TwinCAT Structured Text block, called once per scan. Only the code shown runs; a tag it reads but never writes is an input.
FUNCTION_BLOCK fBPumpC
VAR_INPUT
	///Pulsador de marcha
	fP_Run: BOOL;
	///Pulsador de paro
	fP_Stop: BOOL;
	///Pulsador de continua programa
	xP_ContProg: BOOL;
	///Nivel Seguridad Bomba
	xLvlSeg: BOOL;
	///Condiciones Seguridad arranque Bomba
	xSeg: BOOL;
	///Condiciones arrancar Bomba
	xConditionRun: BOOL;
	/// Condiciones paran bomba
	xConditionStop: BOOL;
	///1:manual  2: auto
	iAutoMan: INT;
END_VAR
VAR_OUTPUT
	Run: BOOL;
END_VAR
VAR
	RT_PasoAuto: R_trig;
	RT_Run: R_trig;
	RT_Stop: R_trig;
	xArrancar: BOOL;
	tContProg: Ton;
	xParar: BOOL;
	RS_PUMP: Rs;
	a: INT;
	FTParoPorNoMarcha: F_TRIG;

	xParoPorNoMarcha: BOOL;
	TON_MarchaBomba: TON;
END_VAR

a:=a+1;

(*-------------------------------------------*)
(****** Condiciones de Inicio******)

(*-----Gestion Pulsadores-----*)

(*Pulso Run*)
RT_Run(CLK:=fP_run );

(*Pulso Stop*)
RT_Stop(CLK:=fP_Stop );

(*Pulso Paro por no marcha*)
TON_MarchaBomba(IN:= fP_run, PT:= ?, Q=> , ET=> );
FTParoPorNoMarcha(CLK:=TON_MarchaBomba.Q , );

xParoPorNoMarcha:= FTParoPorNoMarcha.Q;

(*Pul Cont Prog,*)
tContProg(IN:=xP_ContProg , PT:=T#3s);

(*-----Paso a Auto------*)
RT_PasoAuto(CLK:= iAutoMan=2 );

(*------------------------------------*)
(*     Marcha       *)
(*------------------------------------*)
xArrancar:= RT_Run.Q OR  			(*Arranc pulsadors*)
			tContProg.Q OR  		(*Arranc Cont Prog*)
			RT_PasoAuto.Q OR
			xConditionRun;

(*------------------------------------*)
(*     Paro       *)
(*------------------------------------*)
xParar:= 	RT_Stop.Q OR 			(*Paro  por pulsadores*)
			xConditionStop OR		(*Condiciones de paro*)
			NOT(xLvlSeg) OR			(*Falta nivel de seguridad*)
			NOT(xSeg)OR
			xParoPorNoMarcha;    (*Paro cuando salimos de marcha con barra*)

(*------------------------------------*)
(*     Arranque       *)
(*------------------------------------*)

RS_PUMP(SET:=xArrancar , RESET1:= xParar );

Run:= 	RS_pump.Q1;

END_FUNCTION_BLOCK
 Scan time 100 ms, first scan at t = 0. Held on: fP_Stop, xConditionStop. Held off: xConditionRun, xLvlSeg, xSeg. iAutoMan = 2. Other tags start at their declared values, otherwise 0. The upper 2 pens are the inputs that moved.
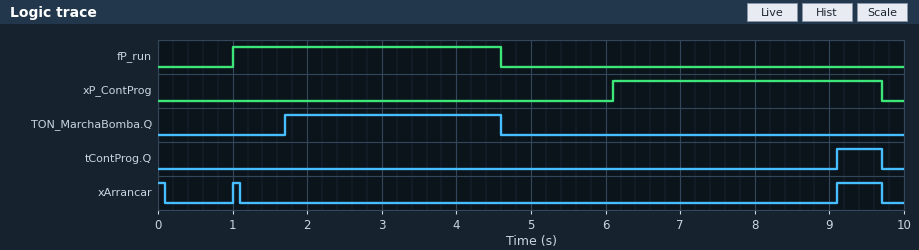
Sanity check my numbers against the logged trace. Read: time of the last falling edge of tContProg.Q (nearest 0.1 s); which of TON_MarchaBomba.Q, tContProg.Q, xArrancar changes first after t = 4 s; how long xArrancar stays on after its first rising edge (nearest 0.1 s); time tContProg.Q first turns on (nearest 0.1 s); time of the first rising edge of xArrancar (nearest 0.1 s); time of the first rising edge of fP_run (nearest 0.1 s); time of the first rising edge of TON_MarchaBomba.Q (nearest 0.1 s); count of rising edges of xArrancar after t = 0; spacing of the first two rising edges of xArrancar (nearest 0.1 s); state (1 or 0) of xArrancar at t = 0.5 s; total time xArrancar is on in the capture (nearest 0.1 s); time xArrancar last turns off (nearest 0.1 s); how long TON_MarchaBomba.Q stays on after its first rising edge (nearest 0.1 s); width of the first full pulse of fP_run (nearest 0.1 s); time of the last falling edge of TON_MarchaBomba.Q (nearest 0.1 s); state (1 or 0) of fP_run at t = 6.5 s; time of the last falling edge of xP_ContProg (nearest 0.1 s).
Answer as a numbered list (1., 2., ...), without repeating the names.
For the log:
1. 9.7 s
2. TON_MarchaBomba.Q
3. 0.1 s
4. 9.1 s
5. 1.0 s
6. 1.0 s
7. 1.7 s
8. 2
9. 8.1 s
10. 0
11. 0.8 s
12. 9.7 s
13. 2.9 s
14. 3.6 s
15. 4.6 s
16. 0
17. 9.7 s
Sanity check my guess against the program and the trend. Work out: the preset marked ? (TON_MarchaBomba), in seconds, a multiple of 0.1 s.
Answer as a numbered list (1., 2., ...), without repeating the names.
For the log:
1. 0.7 s
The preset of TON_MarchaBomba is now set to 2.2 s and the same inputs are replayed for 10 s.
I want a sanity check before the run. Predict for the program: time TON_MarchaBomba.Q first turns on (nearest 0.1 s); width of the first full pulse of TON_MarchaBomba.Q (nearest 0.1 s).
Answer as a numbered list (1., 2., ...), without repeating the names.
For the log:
1. 3.2 s
2. 1.4 s
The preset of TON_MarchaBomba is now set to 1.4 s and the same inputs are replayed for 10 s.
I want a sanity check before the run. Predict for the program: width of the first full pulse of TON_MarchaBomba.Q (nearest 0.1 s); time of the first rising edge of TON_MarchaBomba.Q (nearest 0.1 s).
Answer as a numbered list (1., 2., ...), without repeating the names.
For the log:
1. 2.2 s
2. 2.4 s
